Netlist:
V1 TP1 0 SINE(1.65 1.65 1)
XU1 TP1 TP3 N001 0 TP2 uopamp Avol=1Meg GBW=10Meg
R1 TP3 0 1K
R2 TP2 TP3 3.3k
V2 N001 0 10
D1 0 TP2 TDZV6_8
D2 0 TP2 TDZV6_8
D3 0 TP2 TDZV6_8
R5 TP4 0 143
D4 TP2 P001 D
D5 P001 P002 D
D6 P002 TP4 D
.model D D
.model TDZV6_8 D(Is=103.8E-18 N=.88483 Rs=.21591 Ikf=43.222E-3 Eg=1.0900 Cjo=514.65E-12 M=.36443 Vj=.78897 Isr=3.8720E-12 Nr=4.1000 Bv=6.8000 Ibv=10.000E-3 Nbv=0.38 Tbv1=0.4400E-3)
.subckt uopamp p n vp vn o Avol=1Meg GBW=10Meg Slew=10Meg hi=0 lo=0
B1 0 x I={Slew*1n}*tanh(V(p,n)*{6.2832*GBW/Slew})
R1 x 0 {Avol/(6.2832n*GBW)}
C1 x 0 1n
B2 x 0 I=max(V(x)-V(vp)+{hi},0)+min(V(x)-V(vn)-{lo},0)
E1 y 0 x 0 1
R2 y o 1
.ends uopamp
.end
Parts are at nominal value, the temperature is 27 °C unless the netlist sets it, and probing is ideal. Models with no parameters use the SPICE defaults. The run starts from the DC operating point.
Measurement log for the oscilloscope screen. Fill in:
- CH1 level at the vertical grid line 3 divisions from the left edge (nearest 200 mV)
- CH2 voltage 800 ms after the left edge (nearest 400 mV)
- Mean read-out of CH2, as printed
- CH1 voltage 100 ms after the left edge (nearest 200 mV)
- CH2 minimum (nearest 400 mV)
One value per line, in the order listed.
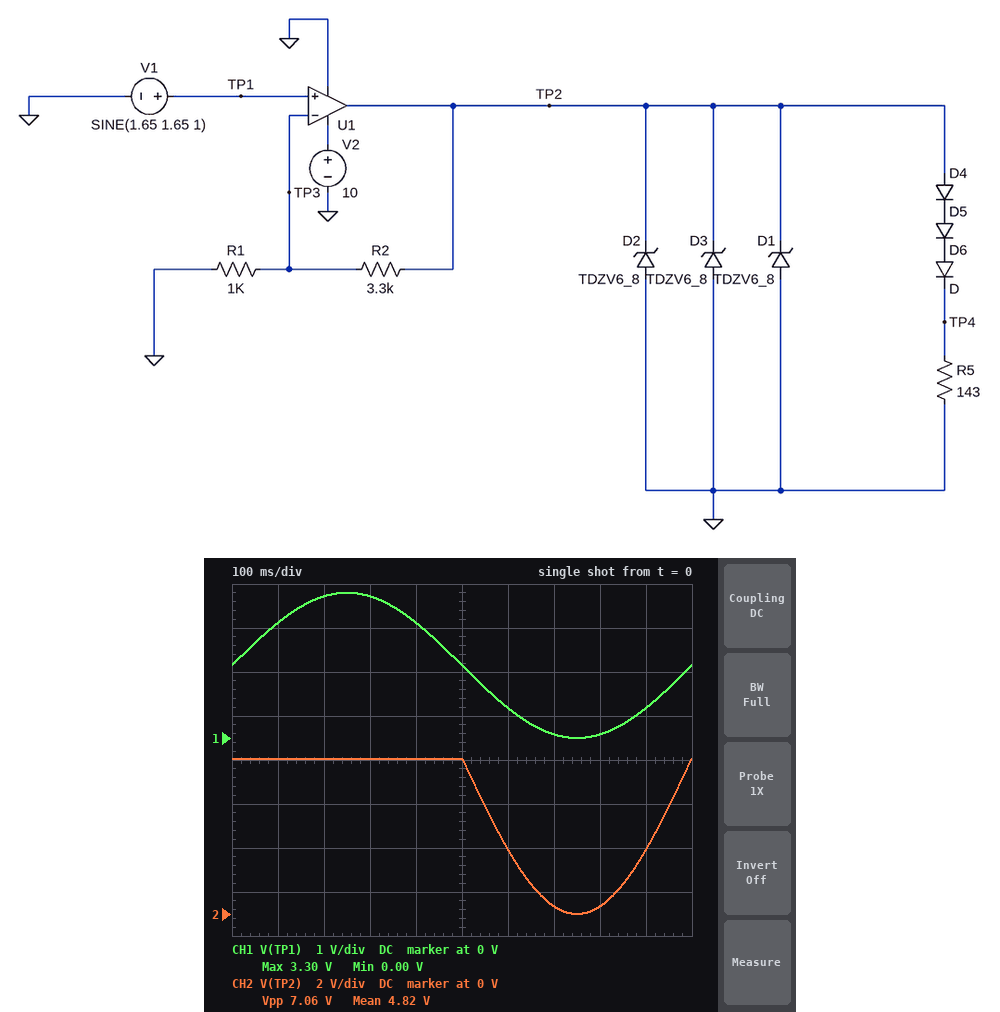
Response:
3.2 V
400 mV
4.82 V
2.6 V
0 V
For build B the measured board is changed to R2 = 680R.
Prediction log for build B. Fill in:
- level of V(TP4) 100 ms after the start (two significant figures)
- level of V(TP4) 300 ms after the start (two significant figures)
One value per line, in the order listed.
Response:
2.2 V
3.2 V
